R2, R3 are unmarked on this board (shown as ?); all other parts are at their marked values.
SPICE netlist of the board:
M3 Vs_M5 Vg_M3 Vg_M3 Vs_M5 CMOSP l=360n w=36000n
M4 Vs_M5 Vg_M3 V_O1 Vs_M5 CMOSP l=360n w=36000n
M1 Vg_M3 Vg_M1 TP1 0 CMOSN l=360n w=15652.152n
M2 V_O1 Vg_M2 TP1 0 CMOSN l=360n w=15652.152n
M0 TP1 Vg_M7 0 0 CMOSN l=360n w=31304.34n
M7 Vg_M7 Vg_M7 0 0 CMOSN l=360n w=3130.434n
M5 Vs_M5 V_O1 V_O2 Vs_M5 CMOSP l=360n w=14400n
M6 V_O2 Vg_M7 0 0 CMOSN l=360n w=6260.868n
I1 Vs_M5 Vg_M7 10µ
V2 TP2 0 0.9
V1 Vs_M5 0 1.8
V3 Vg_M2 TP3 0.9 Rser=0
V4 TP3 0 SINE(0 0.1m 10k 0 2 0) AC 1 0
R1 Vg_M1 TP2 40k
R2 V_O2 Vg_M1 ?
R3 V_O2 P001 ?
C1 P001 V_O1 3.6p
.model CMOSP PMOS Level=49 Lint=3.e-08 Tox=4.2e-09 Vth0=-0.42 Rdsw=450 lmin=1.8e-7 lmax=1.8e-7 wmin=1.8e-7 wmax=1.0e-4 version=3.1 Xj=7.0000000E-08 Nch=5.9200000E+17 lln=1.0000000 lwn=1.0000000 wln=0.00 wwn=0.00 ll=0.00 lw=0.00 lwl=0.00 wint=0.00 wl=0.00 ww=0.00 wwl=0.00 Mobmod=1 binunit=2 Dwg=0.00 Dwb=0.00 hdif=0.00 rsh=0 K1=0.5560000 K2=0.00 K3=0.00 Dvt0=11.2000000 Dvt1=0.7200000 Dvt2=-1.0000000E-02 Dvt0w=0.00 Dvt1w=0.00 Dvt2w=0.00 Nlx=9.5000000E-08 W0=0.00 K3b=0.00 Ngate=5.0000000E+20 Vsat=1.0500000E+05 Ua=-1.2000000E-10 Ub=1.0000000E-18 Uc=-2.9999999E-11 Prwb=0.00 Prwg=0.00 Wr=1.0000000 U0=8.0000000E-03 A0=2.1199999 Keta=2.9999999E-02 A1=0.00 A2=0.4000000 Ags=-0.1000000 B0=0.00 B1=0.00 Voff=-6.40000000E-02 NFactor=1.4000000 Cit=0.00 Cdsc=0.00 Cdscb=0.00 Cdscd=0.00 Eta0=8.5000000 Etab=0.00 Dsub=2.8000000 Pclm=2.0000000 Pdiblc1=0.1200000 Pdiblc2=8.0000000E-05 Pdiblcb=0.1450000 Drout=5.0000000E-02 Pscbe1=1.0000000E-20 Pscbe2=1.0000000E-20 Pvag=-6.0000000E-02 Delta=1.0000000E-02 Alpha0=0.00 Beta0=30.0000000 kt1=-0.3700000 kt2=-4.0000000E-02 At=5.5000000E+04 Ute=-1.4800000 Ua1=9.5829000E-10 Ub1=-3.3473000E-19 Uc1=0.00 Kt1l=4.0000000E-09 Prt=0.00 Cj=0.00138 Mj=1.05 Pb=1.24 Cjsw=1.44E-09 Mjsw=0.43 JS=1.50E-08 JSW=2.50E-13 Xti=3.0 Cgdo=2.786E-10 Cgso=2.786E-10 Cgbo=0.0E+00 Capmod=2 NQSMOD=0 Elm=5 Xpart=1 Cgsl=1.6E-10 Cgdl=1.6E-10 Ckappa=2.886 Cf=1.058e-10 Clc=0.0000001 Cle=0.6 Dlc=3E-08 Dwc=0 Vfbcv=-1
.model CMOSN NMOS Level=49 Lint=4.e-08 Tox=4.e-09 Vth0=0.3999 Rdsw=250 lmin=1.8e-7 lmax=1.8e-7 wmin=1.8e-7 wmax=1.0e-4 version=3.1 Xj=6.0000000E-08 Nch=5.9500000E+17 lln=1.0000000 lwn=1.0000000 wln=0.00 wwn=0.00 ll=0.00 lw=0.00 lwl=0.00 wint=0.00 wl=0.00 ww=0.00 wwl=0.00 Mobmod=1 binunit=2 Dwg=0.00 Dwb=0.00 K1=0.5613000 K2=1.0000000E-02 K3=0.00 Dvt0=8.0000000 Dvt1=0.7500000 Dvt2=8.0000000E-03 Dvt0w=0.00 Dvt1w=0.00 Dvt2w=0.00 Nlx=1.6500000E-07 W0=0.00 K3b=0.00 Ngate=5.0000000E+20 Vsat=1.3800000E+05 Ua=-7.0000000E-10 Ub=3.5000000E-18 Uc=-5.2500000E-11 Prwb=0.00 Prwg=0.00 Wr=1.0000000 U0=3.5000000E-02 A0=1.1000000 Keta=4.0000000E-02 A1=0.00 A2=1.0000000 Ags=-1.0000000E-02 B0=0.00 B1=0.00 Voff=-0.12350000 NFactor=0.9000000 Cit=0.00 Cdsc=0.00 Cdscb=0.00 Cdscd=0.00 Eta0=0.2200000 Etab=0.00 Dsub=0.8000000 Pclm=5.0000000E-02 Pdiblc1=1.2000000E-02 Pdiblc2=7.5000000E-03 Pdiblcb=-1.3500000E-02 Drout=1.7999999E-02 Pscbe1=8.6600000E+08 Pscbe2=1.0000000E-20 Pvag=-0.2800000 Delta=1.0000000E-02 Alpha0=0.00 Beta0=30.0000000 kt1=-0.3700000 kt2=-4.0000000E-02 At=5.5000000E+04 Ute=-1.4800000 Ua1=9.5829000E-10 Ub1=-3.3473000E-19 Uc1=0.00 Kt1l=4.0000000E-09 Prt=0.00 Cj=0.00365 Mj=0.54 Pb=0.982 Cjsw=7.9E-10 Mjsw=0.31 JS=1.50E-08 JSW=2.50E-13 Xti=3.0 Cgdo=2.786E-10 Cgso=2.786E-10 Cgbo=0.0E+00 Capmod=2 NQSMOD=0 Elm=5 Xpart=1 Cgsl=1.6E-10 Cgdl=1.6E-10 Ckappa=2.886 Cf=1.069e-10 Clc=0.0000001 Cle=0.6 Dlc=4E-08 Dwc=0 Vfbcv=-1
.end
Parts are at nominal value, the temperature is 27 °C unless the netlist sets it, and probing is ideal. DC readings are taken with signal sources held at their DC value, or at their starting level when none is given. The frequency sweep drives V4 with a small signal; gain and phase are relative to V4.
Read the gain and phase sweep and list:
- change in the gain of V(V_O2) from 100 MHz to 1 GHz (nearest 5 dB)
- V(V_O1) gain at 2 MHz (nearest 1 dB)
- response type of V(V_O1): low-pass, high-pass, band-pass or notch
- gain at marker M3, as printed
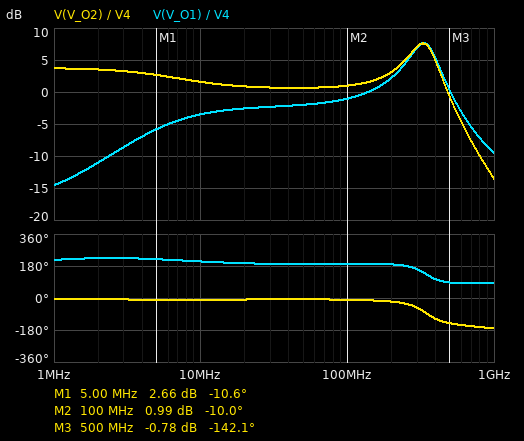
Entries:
-15 dB
-11 dB
band-pass
-0.78 dB
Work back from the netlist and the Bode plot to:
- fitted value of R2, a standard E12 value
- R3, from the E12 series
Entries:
22 kΩ
8.2 kΩ
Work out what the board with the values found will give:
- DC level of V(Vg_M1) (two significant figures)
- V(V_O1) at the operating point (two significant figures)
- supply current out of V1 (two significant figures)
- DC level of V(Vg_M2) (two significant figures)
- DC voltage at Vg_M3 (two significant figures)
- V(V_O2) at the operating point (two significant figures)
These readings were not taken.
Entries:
900 mV
1.2 V
120 µA
900 mV
1.2 V
900 mV
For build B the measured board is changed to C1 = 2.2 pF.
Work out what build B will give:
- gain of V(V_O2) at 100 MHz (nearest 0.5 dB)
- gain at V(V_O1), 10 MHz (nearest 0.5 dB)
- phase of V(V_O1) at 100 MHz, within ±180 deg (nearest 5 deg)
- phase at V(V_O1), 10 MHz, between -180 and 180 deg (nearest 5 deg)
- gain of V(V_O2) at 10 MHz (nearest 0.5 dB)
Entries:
1.0 dB
-5.0 dB
-165 deg
-145 deg
2.5 dB
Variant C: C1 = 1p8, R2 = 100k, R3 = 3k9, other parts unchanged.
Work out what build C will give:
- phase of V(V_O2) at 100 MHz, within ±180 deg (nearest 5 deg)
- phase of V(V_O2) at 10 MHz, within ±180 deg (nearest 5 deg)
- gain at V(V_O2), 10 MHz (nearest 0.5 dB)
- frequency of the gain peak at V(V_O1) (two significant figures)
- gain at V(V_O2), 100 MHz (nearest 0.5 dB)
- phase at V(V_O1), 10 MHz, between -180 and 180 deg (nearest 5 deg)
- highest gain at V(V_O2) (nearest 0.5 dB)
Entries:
-80 deg
-30 deg
9.5 dB
51 MHz
-3.0 dB
-135 deg
11.0 dB
